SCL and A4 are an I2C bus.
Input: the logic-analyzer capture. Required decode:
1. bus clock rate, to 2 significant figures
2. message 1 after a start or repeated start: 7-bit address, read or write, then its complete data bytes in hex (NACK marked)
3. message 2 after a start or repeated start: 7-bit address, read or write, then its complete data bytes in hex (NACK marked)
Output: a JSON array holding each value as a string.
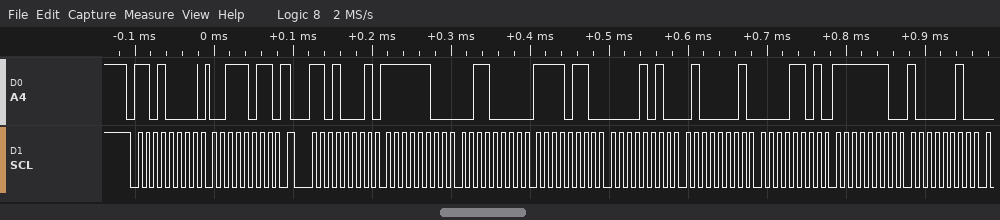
["100 kHz", "0x68 write: 3B", "0x68 read: FC 30 F6 0A 41 0D FE 82"]
